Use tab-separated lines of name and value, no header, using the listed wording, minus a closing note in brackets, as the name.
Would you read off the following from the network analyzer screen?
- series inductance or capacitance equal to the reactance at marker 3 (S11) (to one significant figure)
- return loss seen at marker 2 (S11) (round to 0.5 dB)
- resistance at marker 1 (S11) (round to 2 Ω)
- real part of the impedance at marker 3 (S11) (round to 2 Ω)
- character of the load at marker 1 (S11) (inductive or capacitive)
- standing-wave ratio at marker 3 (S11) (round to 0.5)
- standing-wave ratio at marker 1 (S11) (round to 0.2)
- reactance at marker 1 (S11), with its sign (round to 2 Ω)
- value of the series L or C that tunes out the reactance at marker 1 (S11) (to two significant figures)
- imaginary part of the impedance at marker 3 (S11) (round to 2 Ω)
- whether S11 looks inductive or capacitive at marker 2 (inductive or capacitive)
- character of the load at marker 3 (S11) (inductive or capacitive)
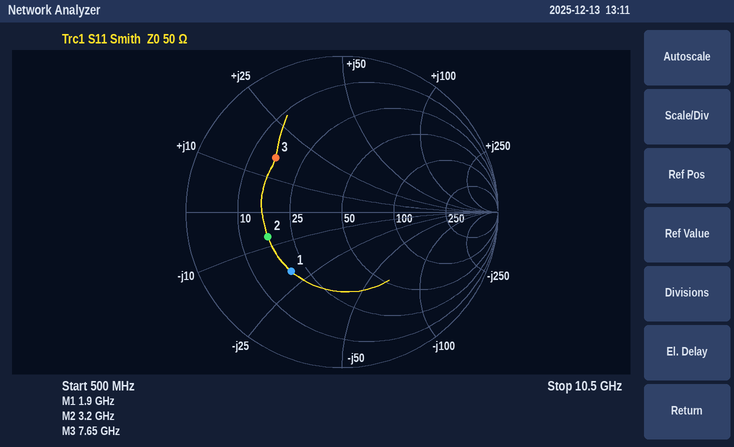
series inductance or capacitance equal to the reactance at marker 3 (S11)	300 pH
return loss seen at marker 2 (S11)	6.0 dB
resistance at marker 1 (S11)	20 Ω
real part of the impedance at marker 3 (S11)	16 Ω
character of the load at marker 1 (S11)	capacitive
standing-wave ratio at marker 3 (S11)	3.5
standing-wave ratio at marker 1 (S11)	3.0
reactance at marker 1 (S11), with its sign	-20 Ω
value of the series L or C that tunes out the reactance at marker 1 (S11)	1.7 nH
imaginary part of the impedance at marker 3 (S11)	+16 Ω
whether S11 looks inductive or capacitive at marker 2	capacitive
character of the load at marker 3 (S11)	inductive
